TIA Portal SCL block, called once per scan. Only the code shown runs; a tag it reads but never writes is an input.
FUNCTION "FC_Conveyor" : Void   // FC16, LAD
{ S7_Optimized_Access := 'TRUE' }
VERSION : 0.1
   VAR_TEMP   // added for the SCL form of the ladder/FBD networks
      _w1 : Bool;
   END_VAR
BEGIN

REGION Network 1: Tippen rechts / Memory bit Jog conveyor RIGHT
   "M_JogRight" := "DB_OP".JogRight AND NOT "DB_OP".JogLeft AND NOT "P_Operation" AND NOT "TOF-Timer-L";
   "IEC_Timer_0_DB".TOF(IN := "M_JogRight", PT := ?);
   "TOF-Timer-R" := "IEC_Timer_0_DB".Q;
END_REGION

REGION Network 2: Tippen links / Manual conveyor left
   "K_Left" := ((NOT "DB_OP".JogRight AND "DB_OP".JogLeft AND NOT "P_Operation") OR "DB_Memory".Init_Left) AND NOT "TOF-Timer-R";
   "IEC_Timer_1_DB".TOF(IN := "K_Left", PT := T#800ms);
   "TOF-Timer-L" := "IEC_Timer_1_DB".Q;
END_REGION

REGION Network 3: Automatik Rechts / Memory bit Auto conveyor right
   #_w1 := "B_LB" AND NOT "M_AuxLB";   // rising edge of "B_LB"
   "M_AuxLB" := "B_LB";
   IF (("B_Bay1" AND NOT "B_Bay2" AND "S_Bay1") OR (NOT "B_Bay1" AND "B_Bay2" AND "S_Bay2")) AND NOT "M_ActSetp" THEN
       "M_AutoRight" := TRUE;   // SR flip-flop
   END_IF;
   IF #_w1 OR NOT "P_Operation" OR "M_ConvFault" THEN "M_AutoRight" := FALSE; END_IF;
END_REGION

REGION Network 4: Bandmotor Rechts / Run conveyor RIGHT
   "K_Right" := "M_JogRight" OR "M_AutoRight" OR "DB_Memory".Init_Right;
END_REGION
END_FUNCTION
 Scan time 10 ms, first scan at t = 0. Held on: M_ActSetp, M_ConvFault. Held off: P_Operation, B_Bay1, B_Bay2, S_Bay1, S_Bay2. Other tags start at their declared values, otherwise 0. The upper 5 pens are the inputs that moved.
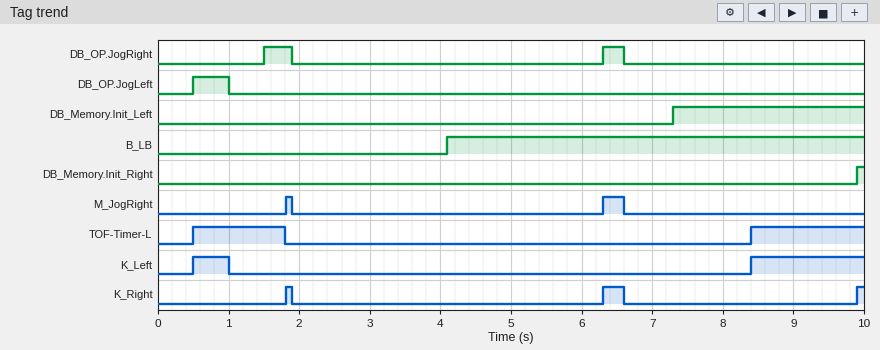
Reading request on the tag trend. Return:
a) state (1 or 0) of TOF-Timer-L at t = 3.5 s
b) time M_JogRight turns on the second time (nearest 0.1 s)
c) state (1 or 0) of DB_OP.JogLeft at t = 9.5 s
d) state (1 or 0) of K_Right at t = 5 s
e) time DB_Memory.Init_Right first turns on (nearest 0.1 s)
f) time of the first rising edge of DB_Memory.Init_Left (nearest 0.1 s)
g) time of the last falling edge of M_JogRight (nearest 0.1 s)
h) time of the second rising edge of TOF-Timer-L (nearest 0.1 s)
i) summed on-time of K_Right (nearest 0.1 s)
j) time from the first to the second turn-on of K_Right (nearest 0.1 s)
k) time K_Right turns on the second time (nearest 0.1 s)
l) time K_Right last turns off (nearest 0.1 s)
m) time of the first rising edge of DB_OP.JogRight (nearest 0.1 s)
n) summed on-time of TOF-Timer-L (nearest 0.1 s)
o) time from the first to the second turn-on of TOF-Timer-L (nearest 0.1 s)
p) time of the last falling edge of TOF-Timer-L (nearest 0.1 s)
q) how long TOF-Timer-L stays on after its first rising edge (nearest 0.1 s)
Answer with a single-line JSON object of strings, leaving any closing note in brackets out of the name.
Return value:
{"state (1 or 0) of TOF-Timer-L at t = 3.5 s": "0", "time M_JogRight turns on the second time": "6.3 s", "state (1 or 0) of DB_OP.JogLeft at t = 9.5 s": "0", "state (1 or 0) of K_Right at t = 5 s": "0", "time DB_Memory.Init_Right first turns on": "9.9 s", "time of the first rising edge of DB_Memory.Init_Left": "7.3 s", "time of the last falling edge of M_JogRight": "6.6 s", "time of the second rising edge of TOF-Timer-L": "8.4 s", "summed on-time of K_Right": "0.5 s", "time from the first to the second turn-on of K_Right": "4.5 s", "time K_Right turns on the second time": "6.3 s", "time K_Right last turns off": "6.6 s", "time of the first rising edge of DB_OP.JogRight": "1.5 s", "summed on-time of TOF-Timer-L": "2.9 s", "time from the first to the second turn-on of TOF-Timer-L": "7.9 s", "time of the last falling edge of TOF-Timer-L": "1.8 s", "how long TOF-Timer-L stays on after its first rising edge": "1.3 s"}
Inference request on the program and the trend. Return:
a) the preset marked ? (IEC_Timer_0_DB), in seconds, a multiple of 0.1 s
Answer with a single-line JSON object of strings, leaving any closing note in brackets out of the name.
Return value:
{"the preset marked ? (IEC_Timer_0_DB), in seconds, a multiple of 0.1 s": "1.8 s"}
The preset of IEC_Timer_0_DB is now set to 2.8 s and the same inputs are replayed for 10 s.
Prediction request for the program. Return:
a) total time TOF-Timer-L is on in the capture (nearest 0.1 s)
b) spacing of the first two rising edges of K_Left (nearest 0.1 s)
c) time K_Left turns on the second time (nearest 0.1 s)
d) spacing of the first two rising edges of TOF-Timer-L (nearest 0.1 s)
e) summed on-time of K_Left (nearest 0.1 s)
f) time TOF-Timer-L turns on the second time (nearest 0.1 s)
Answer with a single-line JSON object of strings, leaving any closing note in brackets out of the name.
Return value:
{"total time TOF-Timer-L is on in the capture": "1.9 s", "spacing of the first two rising edges of K_Left": "8.9 s", "time K_Left turns on the second time": "9.4 s", "spacing of the first two rising edges of TOF-Timer-L": "8.9 s", "summed on-time of K_Left": "1.1 s", "time TOF-Timer-L turns on the second time": "9.4 s"}
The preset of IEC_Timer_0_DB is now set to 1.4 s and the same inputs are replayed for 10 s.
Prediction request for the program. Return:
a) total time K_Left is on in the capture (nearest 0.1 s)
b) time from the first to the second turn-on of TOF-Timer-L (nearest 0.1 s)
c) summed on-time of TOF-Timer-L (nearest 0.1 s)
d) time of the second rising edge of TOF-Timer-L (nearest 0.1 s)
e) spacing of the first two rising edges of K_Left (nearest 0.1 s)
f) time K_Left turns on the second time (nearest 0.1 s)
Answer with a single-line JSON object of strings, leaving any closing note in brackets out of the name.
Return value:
{"total time K_Left is on in the capture": "2.5 s", "time from the first to the second turn-on of TOF-Timer-L": "7.5 s", "summed on-time of TOF-Timer-L": "3.3 s", "time of the second rising edge of TOF-Timer-L": "8.0 s", "spacing of the first two rising edges of K_Left": "7.5 s", "time K_Left turns on the second time": "8.0 s"}
